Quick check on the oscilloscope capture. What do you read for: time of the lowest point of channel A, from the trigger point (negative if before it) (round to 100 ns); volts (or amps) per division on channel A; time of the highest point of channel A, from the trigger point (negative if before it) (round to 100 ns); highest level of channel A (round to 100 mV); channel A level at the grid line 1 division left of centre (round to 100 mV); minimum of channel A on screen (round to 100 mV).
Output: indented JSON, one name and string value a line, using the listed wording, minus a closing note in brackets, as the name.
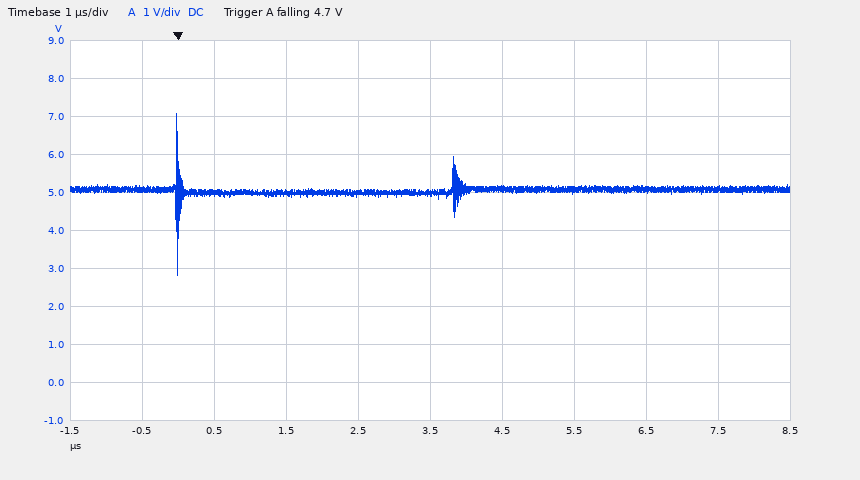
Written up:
{
  "time of the lowest point of channel A, from the trigger point (negative if before it)": "0.0 µs",
  "volts (or amps) per division on channel A": "1 V",
  "time of the highest point of channel A, from the trigger point (negative if before it)": "0.0 µs",
  "highest level of channel A": "7.1 V",
  "channel A level at the grid line 1 division left of centre": "5.0 V",
  "minimum of channel A on screen": "2.8 V"
}
